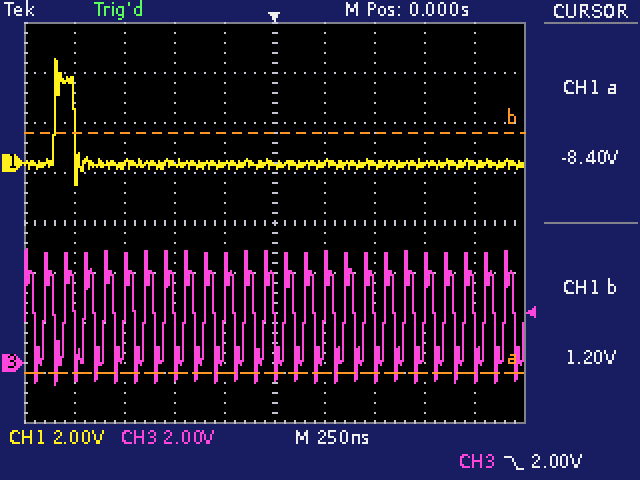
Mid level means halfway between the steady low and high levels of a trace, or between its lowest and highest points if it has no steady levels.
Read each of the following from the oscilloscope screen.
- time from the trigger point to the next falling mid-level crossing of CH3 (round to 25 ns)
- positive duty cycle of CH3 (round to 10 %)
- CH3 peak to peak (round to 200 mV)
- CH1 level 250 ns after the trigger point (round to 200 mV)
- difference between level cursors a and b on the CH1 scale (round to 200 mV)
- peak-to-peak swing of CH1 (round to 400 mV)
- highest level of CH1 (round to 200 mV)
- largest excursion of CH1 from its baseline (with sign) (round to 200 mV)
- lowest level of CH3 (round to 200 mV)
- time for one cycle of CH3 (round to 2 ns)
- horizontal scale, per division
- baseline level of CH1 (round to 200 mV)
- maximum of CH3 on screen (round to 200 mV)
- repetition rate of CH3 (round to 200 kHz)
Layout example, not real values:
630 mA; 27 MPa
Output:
100 ns; 50 %; 5.4 V; 0.0 V; 9.6 V; 5.2 V; 4.2 V; +4.2 V; -800 mV; 100 ns; 250 ns; 0.0 V; 4.6 V; 10.0 MHz
